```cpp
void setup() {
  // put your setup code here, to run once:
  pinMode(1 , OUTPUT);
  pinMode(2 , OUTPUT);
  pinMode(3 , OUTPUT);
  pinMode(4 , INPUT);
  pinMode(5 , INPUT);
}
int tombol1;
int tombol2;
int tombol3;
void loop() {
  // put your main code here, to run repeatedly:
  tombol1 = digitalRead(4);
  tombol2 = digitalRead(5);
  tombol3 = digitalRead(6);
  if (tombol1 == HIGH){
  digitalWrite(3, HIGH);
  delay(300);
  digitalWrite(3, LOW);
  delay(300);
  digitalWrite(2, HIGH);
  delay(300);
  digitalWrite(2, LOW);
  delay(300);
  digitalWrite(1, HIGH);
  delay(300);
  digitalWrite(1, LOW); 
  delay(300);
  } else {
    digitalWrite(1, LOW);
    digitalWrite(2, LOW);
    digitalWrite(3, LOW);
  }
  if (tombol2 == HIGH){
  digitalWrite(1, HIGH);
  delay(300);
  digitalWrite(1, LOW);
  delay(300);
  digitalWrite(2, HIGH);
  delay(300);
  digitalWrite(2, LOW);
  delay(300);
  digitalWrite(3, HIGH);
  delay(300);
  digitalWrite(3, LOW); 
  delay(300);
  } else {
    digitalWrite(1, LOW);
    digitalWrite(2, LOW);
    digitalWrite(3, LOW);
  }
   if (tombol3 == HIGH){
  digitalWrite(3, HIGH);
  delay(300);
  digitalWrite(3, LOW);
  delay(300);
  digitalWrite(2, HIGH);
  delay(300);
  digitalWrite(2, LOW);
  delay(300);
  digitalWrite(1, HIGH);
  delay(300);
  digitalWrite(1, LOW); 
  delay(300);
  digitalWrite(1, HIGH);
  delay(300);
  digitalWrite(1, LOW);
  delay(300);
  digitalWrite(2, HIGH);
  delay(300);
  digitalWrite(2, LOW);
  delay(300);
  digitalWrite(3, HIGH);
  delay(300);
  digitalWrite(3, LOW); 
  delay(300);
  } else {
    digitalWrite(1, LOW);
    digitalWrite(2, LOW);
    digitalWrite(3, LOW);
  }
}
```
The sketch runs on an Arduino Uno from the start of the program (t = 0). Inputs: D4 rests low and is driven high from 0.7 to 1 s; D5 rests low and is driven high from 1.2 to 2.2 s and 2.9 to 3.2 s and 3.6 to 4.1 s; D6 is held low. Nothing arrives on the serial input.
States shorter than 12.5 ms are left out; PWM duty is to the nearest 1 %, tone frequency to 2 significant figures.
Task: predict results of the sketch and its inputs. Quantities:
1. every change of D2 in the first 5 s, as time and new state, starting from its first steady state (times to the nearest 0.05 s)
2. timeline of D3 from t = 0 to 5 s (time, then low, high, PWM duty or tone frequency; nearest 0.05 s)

0 s low; 1.3 s high; 1.6 s low; 3.5 s high; 3.8 s low
0 s low; 0.7 s high; 1 s low; 4.1 s high; 4.4 s low
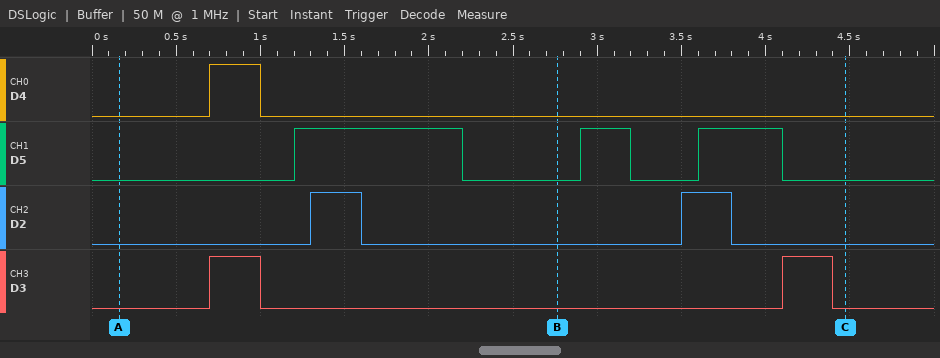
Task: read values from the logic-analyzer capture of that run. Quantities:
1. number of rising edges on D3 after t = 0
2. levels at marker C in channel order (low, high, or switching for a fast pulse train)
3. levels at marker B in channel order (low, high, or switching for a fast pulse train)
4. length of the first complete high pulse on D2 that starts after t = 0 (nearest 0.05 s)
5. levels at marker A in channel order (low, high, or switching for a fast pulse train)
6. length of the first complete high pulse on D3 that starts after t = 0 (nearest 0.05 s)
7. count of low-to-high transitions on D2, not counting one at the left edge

2
D4 low, D5 low, D2 low, D3 low
D4 low, D5 low, D2 low, D3 low
0.30 s
D4 low, D5 low, D2 low, D3 low
0.30 s
2
